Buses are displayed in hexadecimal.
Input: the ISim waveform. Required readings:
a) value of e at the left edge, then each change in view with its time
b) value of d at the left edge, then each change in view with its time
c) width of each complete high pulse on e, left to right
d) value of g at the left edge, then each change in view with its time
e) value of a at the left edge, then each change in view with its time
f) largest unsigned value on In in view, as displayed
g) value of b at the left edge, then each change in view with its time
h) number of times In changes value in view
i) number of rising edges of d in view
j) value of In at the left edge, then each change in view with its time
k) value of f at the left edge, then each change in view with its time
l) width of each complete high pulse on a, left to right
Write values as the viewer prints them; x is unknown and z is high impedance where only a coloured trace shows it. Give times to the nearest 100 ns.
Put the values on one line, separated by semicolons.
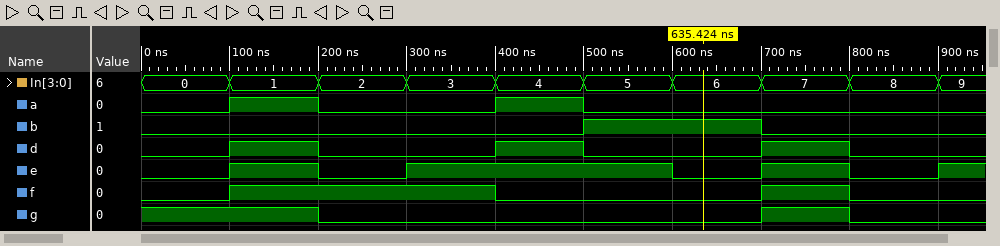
0, 1 at 100 ns, 0 at 200 ns, 1 at 300 ns, 0 at 600 ns, 1 at 700 ns, 0 at 800 ns, 1 at 900 ns; 0, 1 at 100 ns, 0 at 200 ns, 1 at 400 ns, 0 at 500 ns, 1 at 700 ns, 0 at 800 ns; 100 ns, 300 ns, 100 ns; 1, 0 at 200 ns, 1 at 700 ns, 0 at 800 ns; 0, 1 at 100 ns, 0 at 200 ns, 1 at 400 ns, 0 at 500 ns; 9; 0, 1 at 500 ns, 0 at 700 ns; 9; 3; 0, 1 at 100 ns, 2 at 200 ns, 3 at 300 ns, 4 at 400 ns, 5 at 500 ns, 6 at 600 ns, 7 at 700 ns, 8 at 800 ns, 9 at 900 ns; 0, 1 at 100 ns, 0 at 400 ns, 1 at 700 ns, 0 at 800 ns; 100 ns, 100 ns
